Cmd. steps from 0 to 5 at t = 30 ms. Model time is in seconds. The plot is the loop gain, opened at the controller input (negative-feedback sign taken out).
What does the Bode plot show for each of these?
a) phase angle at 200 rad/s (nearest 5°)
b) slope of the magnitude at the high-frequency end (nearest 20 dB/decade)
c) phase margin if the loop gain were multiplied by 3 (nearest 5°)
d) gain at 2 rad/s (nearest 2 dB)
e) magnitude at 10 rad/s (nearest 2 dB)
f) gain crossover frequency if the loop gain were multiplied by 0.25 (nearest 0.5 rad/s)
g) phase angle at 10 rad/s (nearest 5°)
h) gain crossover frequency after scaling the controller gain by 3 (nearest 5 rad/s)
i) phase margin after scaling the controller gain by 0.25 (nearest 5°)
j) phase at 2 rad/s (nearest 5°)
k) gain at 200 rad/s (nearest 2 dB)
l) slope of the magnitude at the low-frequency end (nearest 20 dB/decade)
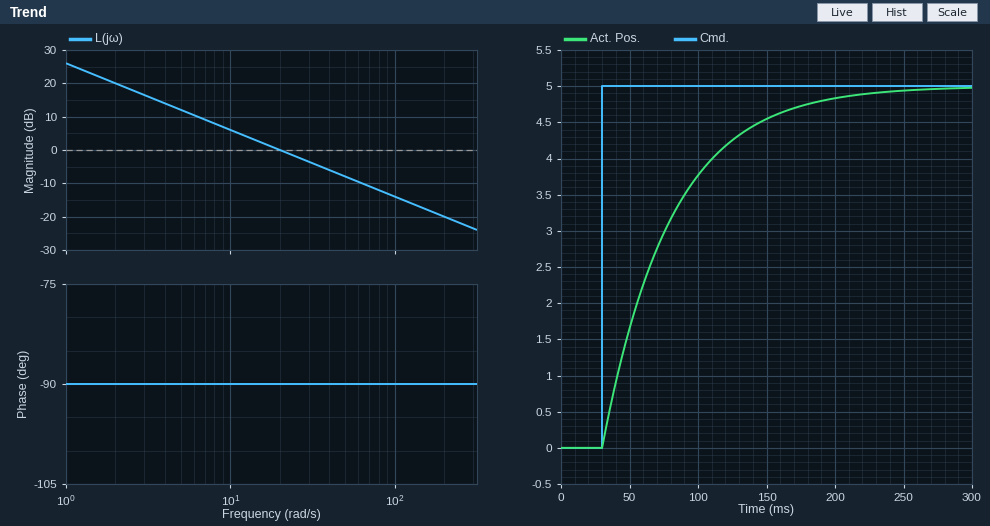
-90°
-20 dB/decade
90°
20 dB
6 dB
5.0 rad/s
-90°
60 rad/s
90°
-90°
-20 dB
-20 dB/decade
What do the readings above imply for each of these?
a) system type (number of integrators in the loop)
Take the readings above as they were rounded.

1
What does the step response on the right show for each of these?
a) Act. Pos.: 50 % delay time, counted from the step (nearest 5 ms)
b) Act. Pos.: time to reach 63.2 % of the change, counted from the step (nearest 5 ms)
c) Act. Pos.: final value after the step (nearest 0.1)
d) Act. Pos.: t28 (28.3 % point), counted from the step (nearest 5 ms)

35 ms
50 ms
5.0
15 ms
